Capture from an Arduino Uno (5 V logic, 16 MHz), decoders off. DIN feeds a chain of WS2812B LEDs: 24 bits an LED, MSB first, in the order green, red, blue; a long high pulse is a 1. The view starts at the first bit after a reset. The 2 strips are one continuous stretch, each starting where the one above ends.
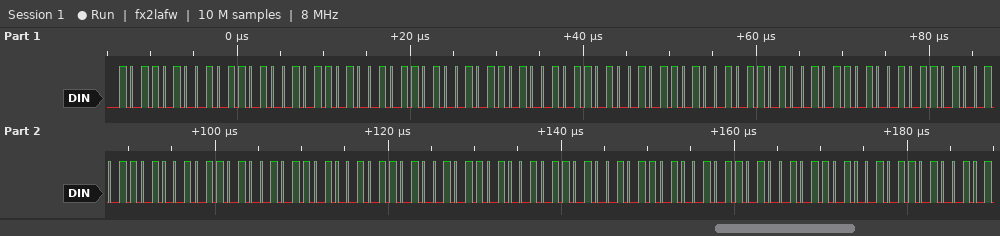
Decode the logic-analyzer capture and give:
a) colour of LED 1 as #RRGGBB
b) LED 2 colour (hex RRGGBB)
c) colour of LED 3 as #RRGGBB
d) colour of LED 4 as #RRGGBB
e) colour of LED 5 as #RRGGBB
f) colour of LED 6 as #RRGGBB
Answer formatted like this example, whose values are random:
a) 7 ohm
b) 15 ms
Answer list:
a) #B4B4B4
b) #B4B4B4
c) #B4B4B4
d) #B4B4B4
e) #B4B4B4
f) #B4B4B4
